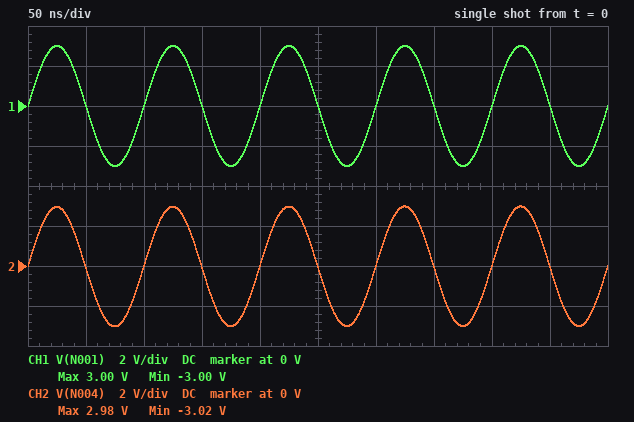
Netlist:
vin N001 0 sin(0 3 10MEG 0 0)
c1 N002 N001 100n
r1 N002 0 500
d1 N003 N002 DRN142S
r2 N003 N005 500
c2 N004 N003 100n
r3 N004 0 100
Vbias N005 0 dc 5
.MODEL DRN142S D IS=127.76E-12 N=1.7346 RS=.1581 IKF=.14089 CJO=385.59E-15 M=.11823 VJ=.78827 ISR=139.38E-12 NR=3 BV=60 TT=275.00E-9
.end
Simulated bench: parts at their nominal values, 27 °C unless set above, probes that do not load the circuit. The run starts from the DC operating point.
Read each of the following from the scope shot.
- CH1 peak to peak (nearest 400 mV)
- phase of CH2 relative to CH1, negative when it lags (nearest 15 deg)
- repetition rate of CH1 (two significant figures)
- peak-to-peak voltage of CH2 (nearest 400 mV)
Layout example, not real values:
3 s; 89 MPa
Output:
6.0 V; 0 deg; 10 MHz; 6.0 V
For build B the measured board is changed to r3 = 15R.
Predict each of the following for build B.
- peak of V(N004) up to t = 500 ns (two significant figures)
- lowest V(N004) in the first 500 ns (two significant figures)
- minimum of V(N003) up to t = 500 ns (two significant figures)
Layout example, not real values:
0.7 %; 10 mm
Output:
3.1 V; -2.9 V; -6.3 mV
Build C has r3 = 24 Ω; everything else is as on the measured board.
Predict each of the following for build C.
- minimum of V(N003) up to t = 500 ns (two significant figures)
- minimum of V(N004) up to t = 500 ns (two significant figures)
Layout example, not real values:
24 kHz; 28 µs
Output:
-50 mV; -2.9 V
